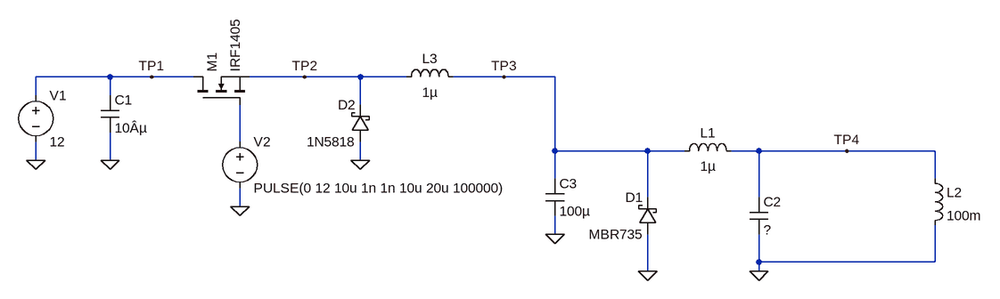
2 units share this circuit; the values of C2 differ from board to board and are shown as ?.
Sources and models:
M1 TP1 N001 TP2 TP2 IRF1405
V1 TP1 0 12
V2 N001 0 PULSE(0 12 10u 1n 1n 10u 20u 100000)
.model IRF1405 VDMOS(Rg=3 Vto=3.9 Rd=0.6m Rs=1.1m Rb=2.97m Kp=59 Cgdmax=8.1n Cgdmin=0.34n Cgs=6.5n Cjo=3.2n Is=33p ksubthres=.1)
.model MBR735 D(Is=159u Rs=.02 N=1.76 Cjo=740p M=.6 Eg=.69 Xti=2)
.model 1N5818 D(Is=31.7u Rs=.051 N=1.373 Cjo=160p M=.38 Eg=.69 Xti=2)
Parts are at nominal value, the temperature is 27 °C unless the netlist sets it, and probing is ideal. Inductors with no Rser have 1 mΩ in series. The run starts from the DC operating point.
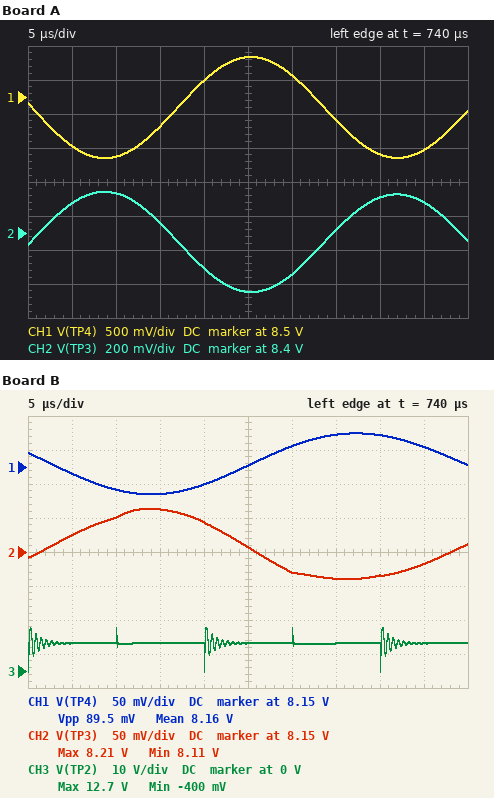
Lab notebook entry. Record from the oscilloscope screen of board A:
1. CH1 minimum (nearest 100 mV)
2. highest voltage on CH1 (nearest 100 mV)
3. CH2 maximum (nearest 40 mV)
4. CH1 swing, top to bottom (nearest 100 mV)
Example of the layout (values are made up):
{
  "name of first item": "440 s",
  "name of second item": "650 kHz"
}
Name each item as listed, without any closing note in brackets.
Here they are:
{
  "CH1 minimum": "7.6 V",
  "highest voltage on CH1": "9.1 V",
  "CH2 maximum": "8.64 V",
  "CH1 swing, top to bottom": "1.5 V"
}
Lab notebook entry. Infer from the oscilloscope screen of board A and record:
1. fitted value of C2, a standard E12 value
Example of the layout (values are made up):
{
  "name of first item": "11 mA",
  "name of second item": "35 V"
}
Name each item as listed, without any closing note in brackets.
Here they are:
{
  "fitted value of C2, a standard E12 value": "39 µF"
}
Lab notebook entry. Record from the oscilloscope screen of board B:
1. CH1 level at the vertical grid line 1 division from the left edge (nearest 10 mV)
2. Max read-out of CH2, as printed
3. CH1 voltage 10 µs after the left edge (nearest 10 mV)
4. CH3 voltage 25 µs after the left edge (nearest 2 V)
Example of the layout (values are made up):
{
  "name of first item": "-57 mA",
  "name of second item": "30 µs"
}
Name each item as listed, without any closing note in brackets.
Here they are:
{
  "CH1 level at the vertical grid line 1 division from the left edge": "8.14 V",
  "Max read-out of CH2, as printed": "8.21 V",
  "CH1 voltage 10 µs after the left edge": "8.12 V",
  "CH3 voltage 25 µs after the left edge": "8 V"
}
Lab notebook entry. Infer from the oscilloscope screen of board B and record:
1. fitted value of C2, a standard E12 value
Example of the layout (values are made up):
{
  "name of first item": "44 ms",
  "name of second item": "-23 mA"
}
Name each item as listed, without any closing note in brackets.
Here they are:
{
  "fitted value of C2, a standard E12 value": "120 µF"
}
